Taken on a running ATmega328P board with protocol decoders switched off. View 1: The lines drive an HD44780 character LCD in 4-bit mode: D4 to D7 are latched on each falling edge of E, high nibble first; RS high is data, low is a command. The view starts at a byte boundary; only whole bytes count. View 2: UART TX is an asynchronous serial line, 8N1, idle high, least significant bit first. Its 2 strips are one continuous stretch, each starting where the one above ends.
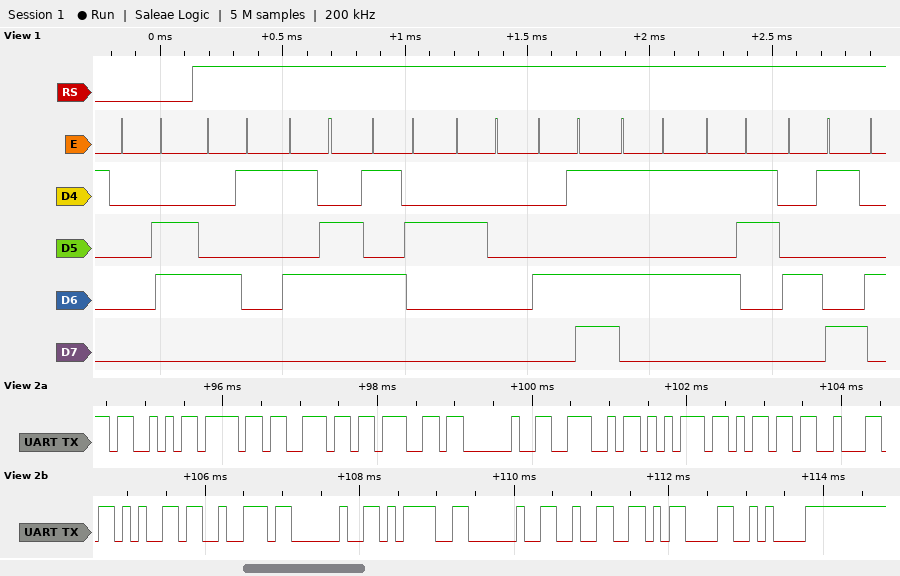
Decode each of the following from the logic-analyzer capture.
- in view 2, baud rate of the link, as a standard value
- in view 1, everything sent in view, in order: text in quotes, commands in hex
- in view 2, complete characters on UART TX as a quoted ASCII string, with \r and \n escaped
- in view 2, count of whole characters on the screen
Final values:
9600 baud
0x06 "AVR MUSI"
"Song Number = 2\r\n"
17
